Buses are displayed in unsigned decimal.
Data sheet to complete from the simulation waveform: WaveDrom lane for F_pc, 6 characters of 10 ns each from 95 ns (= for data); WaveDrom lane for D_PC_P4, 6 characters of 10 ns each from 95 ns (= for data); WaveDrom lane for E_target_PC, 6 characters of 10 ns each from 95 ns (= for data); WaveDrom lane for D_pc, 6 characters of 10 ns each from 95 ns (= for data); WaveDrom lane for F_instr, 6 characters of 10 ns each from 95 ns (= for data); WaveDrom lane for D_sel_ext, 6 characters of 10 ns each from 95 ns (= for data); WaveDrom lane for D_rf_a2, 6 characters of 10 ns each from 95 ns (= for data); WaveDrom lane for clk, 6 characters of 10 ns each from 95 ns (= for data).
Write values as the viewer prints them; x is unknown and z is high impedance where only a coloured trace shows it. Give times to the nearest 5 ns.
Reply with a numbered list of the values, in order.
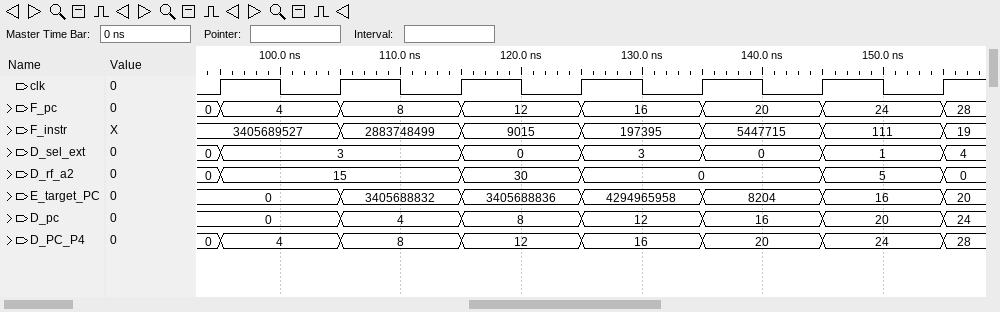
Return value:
1. {name: 'F_pc', wave: '======', data: '4 8 12 16 20 24'}
2. {name: 'D_PC_P4', wave: '======', data: '4 8 12 16 20 24'}
3. {name: 'E_target_PC', wave: '======', data: '0 3405688832 3405688836 4294965958 8204 16'}
4. {name: 'D_pc', wave: '======', data: '0 4 8 12 16 20'}
5. {name: 'F_instr', wave: '======', data: '3405689527 2883748499 9015 197395 5447715 111'}
6. {name: 'D_sel_ext', wave: '=.====', data: '3 0 3 0 1'}
7. {name: 'D_rf_a2', wave: '=.==.=', data: '15 30 0 5'}
8. {name: 'clk', wave: 'p.....'}
